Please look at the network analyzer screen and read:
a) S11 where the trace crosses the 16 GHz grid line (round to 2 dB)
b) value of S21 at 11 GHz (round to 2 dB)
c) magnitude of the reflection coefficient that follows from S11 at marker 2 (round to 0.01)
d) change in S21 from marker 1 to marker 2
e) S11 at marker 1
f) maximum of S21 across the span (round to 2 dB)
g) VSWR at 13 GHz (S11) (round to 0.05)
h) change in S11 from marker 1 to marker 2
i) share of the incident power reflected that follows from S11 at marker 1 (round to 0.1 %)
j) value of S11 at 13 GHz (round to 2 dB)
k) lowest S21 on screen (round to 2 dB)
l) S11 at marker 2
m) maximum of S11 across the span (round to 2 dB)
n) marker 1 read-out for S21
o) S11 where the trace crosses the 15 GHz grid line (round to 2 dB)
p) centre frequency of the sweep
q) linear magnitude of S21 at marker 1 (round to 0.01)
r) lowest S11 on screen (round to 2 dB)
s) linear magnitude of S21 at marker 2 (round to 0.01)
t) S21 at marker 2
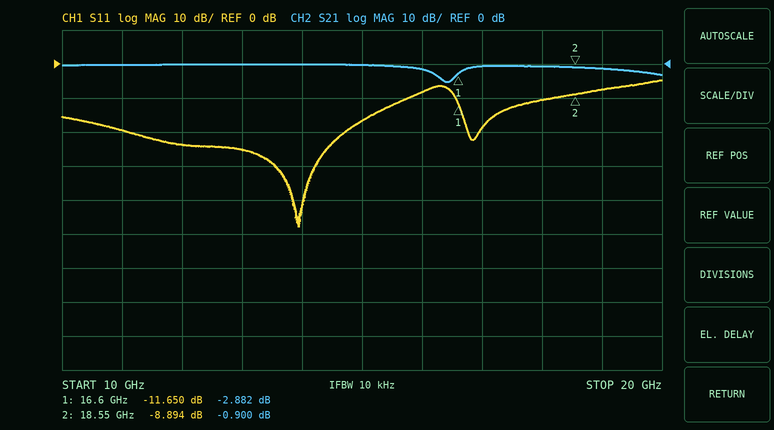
-8 dB
0 dB
0.36
1.982 dB
-11.650 dB
0 dB
1.10
2.756 dB
6.8 %
-26 dB
-6 dB
-8.894 dB
-4 dB
-2.882 dB
-16 dB
15 GHz
0.72
-48 dB
0.90
-0.900 dB
